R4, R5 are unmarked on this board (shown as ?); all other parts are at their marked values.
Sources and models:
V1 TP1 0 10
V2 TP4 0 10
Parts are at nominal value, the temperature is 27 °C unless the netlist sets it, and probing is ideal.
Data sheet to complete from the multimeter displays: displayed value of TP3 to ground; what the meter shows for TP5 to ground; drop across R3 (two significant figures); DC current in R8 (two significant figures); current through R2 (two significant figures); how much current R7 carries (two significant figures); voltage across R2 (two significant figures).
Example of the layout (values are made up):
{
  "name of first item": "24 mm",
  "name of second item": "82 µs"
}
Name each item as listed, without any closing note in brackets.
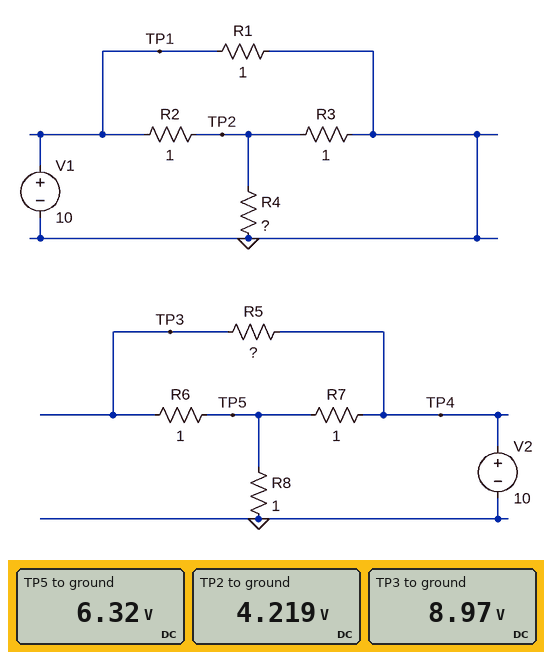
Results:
{
  "displayed value of TP3 to ground": "8.97 V",
  "what the meter shows for TP5 to ground": "6.32 V",
  "drop across R3": "4.2 V",
  "DC current in R8": "6.3 A",
  "current through R2": "5.8 A",
  "how much current R7 carries": "3.7 A",
  "voltage across R2": "5.8 V"
}
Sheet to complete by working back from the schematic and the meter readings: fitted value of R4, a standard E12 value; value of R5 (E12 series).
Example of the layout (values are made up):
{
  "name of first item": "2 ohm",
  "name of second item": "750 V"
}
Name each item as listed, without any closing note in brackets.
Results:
{
  "fitted value of R4, a standard E12 value": "2.7 Ω",
  "value of R5": "0.39 Ω"
}
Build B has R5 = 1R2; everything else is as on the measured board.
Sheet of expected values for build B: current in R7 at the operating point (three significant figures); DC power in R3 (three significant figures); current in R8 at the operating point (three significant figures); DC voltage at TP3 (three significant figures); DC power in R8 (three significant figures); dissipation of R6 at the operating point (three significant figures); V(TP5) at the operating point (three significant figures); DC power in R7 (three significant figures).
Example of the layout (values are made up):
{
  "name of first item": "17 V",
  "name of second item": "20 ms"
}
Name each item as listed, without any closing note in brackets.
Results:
{
  "current in R7 at the operating point": "4.07 A",
  "DC power in R3": "17.8 W",
  "current in R8 at the operating point": "5.93 A",
  "DC voltage at TP3": "7.78 V",
  "DC power in R8": "35.1 W",
  "dissipation of R6 at the operating point": "3.43 W",
  "V(TP5) at the operating point": "5.93 V",
  "DC power in R7": "16.6 W"
}
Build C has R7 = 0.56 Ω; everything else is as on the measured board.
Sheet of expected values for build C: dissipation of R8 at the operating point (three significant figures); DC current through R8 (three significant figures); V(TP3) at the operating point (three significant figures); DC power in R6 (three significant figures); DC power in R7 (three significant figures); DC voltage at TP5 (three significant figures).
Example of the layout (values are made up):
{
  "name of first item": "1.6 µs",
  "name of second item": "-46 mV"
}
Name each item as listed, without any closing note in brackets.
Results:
{
  "dissipation of R8 at the operating point": "51.1 W",
  "DC current through R8": "7.15 A",
  "V(TP3) at the operating point": "9.20 V",
  "DC power in R6": "4.21 W",
  "DC power in R7": "14.5 W",
  "DC voltage at TP5": "7.15 V"
}
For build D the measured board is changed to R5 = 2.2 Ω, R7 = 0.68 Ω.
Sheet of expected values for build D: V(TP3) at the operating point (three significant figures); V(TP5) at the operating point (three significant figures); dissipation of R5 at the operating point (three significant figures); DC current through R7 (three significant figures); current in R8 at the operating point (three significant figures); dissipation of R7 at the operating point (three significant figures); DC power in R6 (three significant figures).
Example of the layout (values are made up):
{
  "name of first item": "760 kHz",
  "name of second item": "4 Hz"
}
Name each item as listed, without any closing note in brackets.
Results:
{
  "V(TP3) at the operating point": "7.53 V",
  "V(TP5) at the operating point": "6.41 V",
  "dissipation of R5 at the operating point": "2.77 W",
  "DC current through R7": "5.28 A",
  "current in R8 at the operating point": "6.41 A",
  "dissipation of R7 at the operating point": "19.0 W",
  "DC power in R6": "1.26 W"
}
